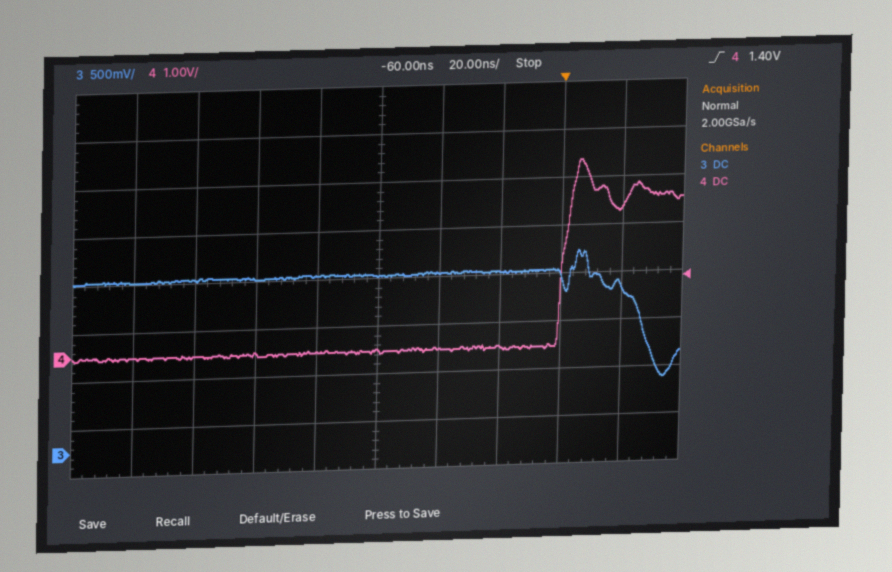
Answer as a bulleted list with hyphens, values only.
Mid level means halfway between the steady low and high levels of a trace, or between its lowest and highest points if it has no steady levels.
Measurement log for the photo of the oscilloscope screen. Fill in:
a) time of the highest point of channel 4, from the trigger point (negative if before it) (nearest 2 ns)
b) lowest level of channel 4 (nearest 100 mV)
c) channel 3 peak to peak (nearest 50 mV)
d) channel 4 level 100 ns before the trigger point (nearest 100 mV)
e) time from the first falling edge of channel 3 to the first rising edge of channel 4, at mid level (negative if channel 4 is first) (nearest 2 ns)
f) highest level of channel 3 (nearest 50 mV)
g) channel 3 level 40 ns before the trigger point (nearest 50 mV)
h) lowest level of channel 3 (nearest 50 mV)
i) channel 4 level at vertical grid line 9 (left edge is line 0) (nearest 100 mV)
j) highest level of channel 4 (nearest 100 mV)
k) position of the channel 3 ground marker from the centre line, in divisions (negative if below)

- +6 ns
- -100 mV
- 1.35 V
- 0.0 V
- -26 ns
- 2.00 V
- 1.80 V
- 650 mV
- 2.9 V
- 3.9 V
- -3.5 div
